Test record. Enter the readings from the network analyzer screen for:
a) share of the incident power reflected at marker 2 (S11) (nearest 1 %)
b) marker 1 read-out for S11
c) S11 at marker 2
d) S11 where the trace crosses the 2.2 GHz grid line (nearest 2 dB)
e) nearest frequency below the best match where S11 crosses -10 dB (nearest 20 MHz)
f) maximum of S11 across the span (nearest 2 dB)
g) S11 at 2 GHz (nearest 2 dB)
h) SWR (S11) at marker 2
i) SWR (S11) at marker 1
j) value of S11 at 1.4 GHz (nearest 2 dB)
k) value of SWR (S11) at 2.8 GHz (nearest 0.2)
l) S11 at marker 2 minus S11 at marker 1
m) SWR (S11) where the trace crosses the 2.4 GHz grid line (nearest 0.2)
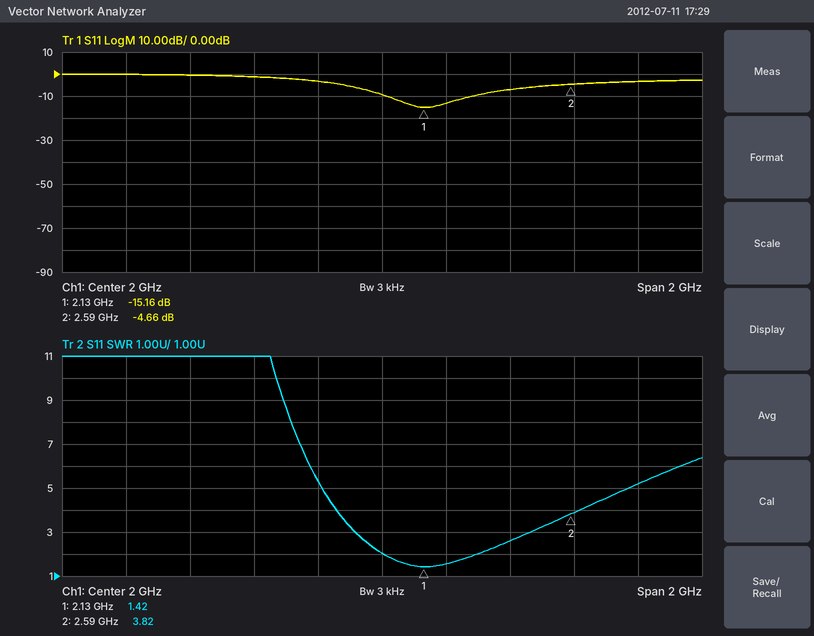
34 %
-15.16 dB
-4.66 dB
-14 dB
2.02 GHz
0 dB
-10 dB
3.82
1.42
0 dB
5.2
10.50 dB
2.6
